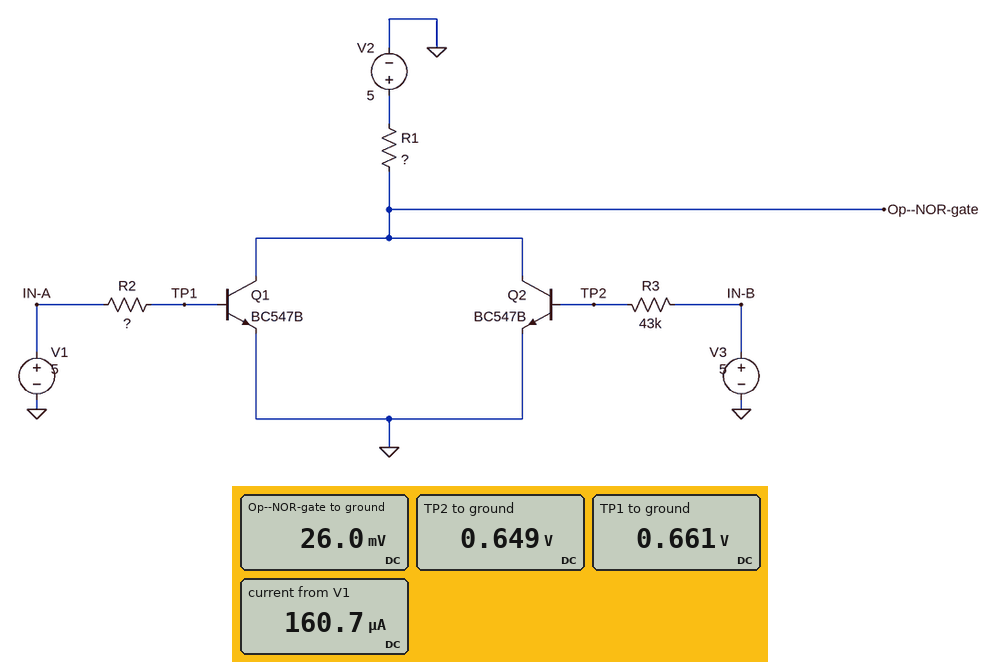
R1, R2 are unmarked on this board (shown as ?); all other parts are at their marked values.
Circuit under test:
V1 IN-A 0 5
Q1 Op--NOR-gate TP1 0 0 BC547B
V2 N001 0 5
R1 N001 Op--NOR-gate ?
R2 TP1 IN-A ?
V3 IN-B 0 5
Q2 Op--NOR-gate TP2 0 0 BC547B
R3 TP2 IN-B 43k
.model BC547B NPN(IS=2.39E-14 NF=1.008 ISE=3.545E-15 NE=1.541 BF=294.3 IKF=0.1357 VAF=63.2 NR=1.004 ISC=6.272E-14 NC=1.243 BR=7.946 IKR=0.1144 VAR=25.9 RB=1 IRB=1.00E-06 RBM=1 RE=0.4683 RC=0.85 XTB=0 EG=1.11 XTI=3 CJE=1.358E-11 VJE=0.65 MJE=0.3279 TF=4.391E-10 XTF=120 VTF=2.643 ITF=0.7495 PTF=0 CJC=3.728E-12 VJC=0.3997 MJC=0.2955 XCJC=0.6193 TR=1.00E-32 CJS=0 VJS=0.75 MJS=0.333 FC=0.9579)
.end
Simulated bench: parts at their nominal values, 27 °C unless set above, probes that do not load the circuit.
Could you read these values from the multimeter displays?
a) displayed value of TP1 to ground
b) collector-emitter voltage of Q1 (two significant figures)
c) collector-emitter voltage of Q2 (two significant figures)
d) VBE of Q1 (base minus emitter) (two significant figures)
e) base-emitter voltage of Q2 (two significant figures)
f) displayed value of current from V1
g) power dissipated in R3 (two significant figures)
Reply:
0.661 V
26 mV
26 mV
660 mV
650 mV
160.7 µA
440 µW
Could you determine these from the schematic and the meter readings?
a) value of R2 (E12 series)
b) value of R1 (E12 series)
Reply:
27 kΩ
2.7 kΩ
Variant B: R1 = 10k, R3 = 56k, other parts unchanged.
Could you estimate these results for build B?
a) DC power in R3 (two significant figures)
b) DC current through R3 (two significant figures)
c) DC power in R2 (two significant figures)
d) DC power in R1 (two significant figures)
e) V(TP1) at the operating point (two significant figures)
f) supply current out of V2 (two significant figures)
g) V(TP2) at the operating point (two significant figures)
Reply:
340 µW
78 µA
700 µW
2.5 mW
650 mV
500 µA
630 mV
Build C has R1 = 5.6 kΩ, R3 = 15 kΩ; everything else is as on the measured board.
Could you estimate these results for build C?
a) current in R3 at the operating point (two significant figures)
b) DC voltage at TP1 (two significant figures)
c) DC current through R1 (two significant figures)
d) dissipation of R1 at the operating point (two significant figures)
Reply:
290 µA
650 mV
890 µA
4.4 mW
